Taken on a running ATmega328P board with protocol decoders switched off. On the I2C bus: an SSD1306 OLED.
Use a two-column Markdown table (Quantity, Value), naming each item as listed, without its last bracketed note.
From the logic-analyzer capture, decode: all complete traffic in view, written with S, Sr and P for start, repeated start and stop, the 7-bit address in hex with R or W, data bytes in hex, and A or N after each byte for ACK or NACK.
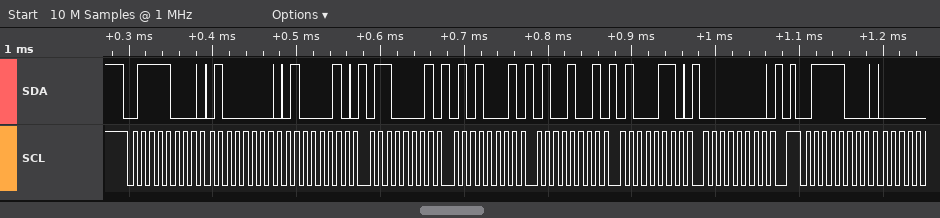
| Quantity | Value |
|---|---|
| all complete traffic in view, written with S, Sr and P for start, repeated start and stop, the 7-bit address in hex with R or W, data bytes in hex, and A or N after each byte for ACK or NACK | S 3CW A 40 A 42 A 61 A 51 A 49 A 46 A 00 A P S 3CW A |
